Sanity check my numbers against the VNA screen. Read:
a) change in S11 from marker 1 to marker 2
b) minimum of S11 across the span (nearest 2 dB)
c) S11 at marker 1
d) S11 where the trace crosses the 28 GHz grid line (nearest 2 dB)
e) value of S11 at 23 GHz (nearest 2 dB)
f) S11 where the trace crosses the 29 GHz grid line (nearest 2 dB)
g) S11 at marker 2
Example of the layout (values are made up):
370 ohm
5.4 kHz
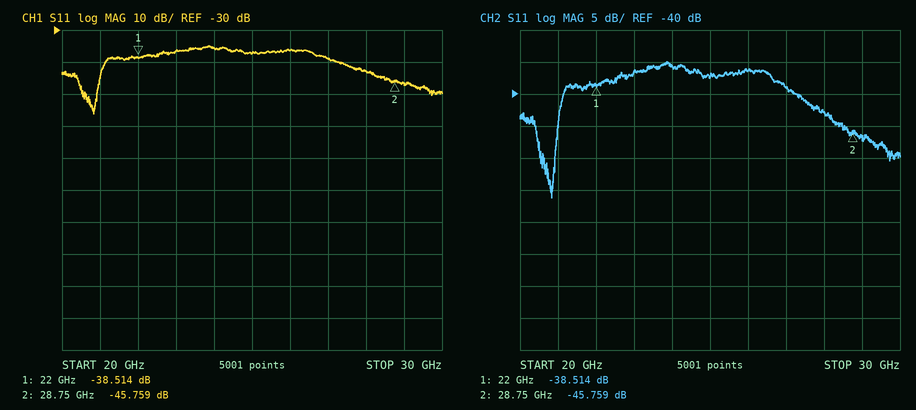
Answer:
-7.245 dB
-56 dB
-38.514 dB
-42 dB
-36 dB
-46 dB
-45.759 dB
